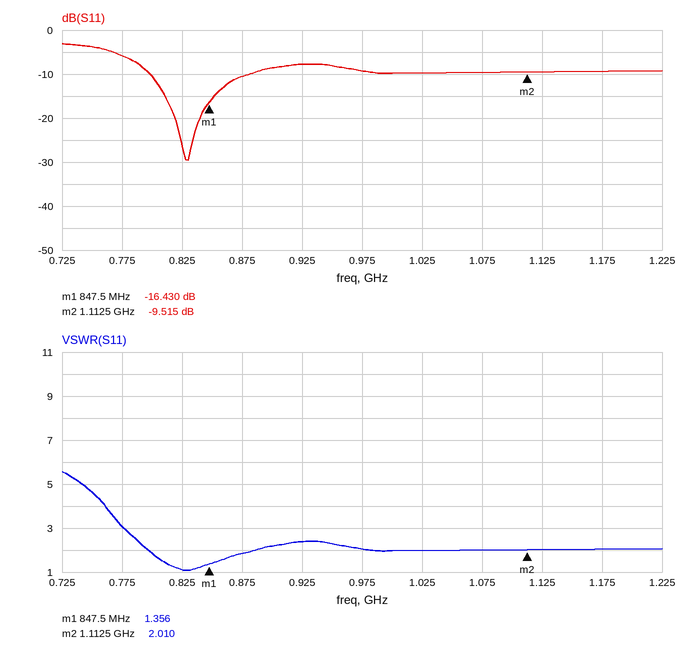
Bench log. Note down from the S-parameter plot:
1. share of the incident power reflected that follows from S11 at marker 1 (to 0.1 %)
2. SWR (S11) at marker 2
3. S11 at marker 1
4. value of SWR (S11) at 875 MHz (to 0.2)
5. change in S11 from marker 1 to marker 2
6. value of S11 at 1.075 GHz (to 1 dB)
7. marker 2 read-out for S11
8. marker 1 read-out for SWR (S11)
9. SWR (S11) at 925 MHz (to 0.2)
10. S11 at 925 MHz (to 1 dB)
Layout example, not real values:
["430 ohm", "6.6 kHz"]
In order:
["2.3 %", "2.010", "-16.430 dB", "1.8", "6.915 dB", "-10 dB", "-9.515 dB", "1.356", "2.4", "-8 dB"]
